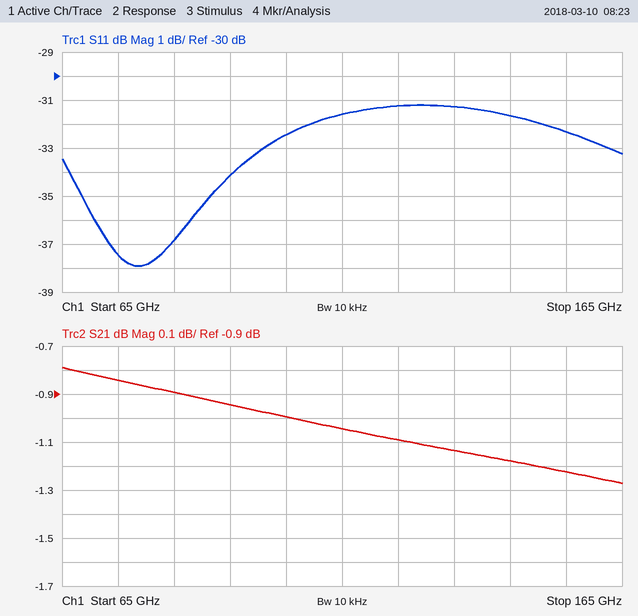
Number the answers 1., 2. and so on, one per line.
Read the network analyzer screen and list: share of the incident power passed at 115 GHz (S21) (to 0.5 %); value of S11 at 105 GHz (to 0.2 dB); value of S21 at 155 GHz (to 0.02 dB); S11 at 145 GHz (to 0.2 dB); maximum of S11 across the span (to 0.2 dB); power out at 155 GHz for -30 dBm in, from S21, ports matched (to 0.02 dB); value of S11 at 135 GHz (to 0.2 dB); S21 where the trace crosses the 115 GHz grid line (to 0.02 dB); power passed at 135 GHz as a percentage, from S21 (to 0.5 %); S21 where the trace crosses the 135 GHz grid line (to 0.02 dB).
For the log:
1. 78.5 %
2. -32.4 dB
3. -1.22 dB
4. -31.6 dB
5. -31.2 dB
6. -31.22 dBm
7. -31.2 dB
8. -1.04 dB
9. 77.0 %
10. -1.14 dB
